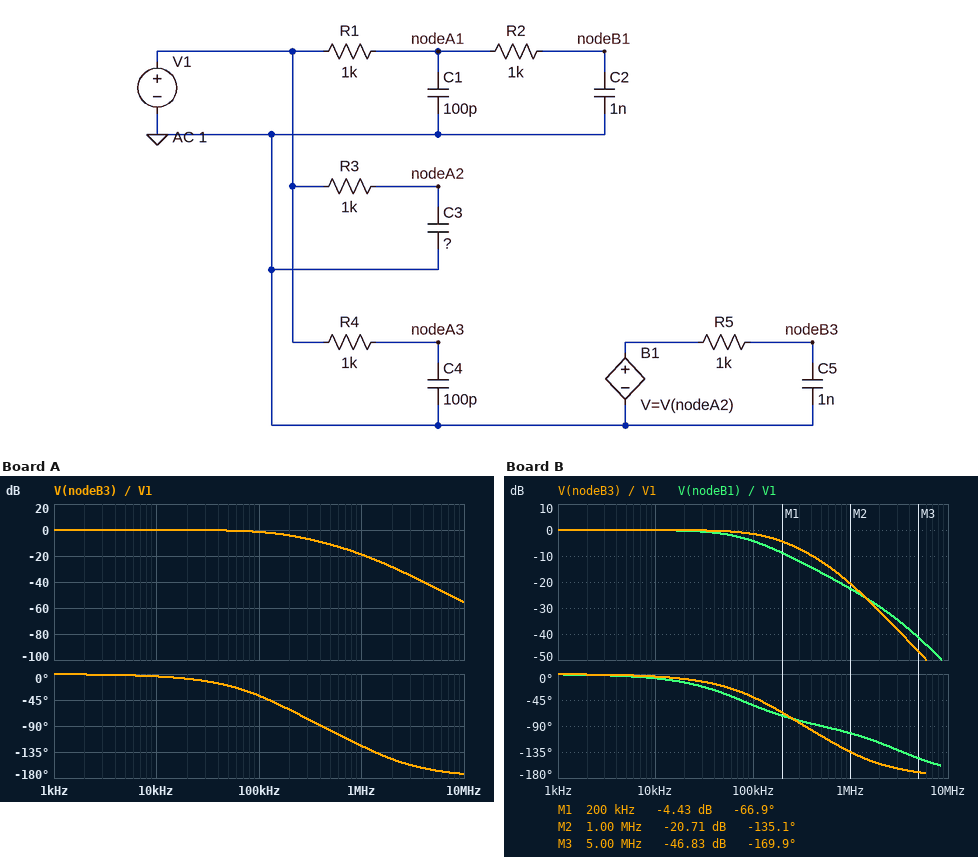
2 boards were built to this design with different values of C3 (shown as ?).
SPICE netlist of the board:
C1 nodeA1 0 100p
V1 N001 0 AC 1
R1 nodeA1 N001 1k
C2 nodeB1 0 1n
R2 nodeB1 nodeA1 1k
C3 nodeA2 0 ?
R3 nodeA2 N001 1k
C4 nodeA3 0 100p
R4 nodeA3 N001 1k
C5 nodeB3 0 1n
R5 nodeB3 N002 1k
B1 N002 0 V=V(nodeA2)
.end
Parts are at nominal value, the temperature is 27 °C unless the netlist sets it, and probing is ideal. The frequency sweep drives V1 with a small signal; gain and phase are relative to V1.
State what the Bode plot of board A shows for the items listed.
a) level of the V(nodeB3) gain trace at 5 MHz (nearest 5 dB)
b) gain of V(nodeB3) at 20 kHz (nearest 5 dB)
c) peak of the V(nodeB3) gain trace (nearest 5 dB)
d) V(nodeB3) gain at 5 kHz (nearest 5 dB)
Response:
-45 dB
0 dB
0 dB
0 dB
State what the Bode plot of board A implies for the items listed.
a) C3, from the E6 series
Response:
150 pF
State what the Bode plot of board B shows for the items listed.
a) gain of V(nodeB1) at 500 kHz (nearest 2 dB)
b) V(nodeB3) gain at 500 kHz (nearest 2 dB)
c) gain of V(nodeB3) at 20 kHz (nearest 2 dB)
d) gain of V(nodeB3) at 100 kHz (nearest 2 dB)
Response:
-16 dB
-12 dB
0 dB
-2 dB
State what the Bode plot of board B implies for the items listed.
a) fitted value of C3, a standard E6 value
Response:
220 pF
